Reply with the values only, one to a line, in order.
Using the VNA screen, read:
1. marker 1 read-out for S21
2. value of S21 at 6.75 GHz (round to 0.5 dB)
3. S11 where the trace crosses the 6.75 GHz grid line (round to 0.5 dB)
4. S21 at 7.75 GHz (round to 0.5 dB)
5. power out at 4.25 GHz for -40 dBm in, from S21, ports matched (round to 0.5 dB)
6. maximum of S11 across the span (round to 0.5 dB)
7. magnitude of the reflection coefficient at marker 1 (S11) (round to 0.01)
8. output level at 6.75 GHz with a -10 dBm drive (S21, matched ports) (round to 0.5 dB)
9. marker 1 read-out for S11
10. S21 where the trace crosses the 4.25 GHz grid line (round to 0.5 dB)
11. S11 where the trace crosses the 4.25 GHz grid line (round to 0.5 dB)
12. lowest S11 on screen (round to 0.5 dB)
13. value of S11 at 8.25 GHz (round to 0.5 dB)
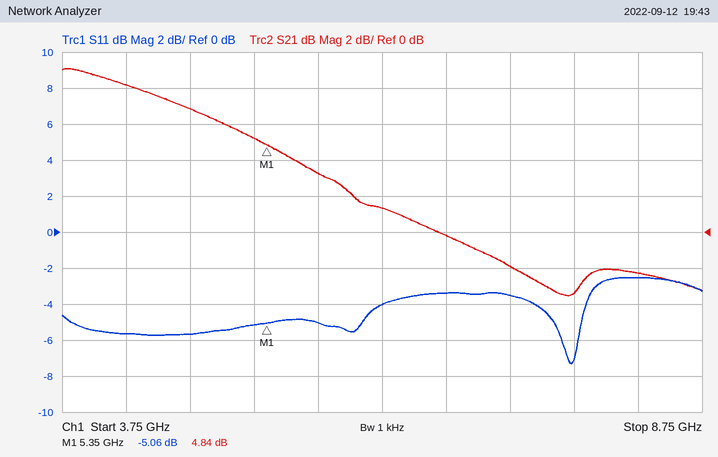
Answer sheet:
4.84 dB
0.0 dB
-3.5 dB
-3.5 dB
-32.0 dBm
-2.5 dB
0.56
-10.0 dBm
-5.06 dB
8.0 dB
-5.5 dB
-7.5 dB
-2.5 dB
